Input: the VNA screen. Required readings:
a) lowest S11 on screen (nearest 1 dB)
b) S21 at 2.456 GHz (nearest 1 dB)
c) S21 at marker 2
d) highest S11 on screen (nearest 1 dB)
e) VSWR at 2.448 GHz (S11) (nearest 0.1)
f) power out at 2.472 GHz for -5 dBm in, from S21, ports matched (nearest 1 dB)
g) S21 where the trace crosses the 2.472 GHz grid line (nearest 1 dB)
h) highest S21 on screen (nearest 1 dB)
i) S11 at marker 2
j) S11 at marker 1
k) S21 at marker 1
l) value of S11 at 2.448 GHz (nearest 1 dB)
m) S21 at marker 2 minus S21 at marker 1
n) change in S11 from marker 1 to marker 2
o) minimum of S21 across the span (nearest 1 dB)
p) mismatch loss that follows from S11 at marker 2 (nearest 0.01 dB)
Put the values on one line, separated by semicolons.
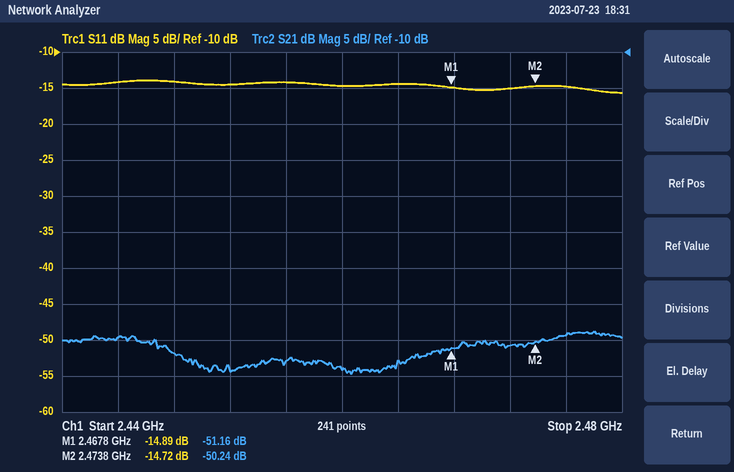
-16 dB; -53 dB; -50.24 dB; -14 dB; 1.5; -56 dBm; -51 dB; -49 dB; -14.72 dB; -14.89 dB; -51.16 dB; -14 dB; 0.92 dB; 0.17 dB; -55 dB; 0.15 dB
